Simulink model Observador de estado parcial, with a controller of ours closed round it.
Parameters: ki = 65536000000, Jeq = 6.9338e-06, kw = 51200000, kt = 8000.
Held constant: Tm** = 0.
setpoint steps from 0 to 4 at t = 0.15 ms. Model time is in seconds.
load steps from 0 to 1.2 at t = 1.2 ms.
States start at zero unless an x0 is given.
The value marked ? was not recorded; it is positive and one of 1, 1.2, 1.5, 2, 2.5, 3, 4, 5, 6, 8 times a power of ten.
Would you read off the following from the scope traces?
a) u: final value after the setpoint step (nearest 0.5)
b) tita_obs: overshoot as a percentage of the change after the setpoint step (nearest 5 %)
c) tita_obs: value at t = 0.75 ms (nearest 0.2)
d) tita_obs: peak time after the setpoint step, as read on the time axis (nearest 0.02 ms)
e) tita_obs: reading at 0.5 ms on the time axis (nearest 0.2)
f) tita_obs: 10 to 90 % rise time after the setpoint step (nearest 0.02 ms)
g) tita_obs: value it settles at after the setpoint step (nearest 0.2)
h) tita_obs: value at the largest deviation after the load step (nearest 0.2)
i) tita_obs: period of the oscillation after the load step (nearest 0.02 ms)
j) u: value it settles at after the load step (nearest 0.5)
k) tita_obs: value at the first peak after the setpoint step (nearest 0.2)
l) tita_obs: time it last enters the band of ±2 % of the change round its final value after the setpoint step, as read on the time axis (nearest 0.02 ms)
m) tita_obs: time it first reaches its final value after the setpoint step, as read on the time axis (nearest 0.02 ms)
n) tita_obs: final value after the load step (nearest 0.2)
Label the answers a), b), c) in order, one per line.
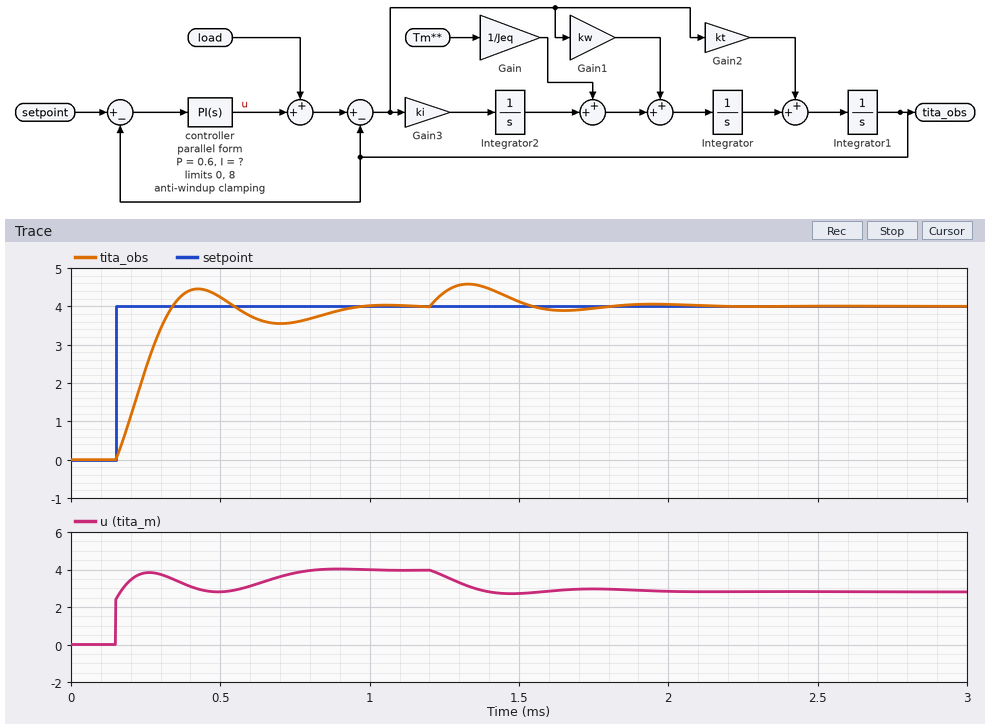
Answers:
a) 4.0
b) 10 %
c) 3.6
d) 0.42 ms
e) 4.2
f) 0.14 ms
g) 4.0
h) 4.6
i) 0.62 ms
j) 3.0
k) 4.4
l) 0.92 ms
m) 0.34 ms
n) 4.0
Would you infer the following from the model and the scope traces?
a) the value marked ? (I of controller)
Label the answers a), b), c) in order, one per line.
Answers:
a) 10000
